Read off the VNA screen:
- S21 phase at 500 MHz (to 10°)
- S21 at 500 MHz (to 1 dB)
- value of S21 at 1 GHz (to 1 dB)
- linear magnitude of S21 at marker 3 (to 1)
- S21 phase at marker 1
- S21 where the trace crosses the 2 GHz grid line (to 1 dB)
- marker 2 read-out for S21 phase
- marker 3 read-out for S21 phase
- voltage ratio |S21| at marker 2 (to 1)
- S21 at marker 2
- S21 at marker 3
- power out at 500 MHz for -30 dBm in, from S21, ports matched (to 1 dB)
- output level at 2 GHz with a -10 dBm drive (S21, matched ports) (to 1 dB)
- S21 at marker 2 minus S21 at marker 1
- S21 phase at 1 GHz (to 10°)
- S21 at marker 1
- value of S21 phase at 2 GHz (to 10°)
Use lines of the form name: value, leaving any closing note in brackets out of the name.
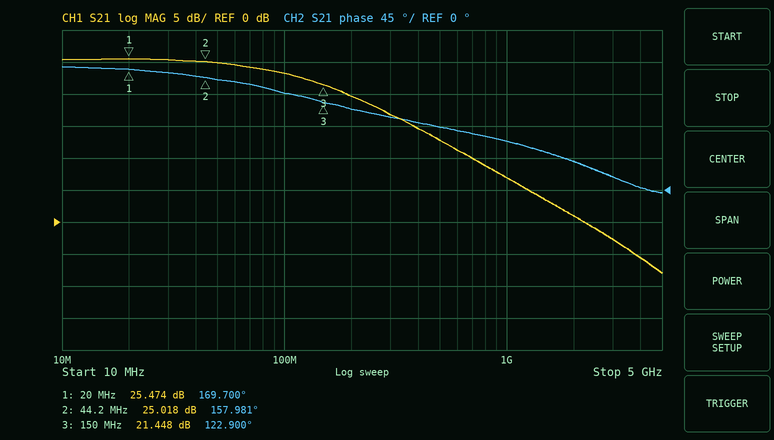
S21 phase at 500 MHz: 90°
S21 at 500 MHz: 13 dB
value of S21 at 1 GHz: 7 dB
linear magnitude of S21 at marker 3: 12
S21 phase at marker 1: 169.700°
S21 where the trace crosses the 2 GHz grid line: 1 dB
marker 2 read-out for S21 phase: 157.981°
marker 3 read-out for S21 phase: 122.900°
voltage ratio |S21| at marker 2: 18
S21 at marker 2: 25.018 dB
S21 at marker 3: 21.448 dB
power out at 500 MHz for -30 dBm in, from S21, ports matched: -17 dBm
output level at 2 GHz with a -10 dBm drive (S21, matched ports): -9 dBm
S21 at marker 2 minus S21 at marker 1: -0.456 dB
S21 phase at 1 GHz: 70°
S21 at marker 1: 25.474 dB
value of S21 phase at 2 GHz: 40°
